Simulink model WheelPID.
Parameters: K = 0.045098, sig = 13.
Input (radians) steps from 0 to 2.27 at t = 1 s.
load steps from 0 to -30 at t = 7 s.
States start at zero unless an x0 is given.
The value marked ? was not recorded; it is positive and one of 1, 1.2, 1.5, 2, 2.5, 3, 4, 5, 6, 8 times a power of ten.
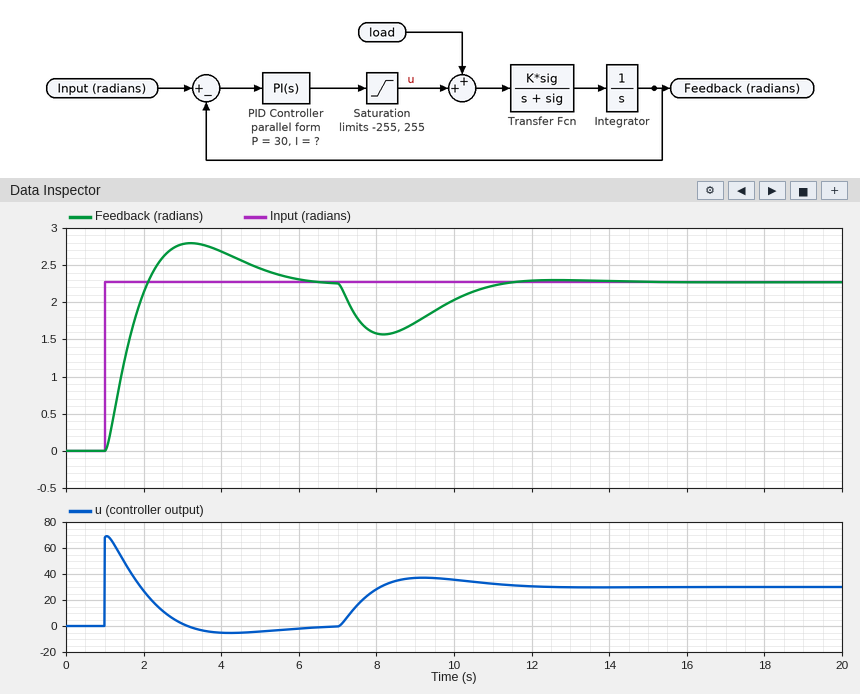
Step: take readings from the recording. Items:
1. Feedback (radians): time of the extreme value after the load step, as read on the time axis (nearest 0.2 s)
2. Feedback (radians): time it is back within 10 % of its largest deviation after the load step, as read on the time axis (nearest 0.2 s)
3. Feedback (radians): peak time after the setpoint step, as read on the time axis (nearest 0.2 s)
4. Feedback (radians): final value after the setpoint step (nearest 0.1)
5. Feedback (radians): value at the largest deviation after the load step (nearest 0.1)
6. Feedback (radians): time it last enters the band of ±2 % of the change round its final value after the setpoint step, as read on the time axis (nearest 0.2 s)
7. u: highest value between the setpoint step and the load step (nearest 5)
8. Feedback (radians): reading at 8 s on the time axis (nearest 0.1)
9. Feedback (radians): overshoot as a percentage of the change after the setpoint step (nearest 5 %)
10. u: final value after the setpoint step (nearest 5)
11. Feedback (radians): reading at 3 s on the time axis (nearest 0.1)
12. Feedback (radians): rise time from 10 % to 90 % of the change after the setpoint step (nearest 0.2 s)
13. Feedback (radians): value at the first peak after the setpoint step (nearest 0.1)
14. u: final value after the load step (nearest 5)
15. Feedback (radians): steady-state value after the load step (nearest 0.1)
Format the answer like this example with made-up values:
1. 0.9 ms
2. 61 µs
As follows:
1. 8.2 s
2. 10.8 s
3. 3.2 s
4. 2.3
5. 1.6
6. 6.0 s
7. 70
8. 1.6
9. 25 %
10. 0
11. 2.8
12. 0.8 s
13. 2.8
14. 30
15. 2.3
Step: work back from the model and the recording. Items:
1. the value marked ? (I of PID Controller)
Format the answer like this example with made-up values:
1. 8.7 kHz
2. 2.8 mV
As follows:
1. 20
